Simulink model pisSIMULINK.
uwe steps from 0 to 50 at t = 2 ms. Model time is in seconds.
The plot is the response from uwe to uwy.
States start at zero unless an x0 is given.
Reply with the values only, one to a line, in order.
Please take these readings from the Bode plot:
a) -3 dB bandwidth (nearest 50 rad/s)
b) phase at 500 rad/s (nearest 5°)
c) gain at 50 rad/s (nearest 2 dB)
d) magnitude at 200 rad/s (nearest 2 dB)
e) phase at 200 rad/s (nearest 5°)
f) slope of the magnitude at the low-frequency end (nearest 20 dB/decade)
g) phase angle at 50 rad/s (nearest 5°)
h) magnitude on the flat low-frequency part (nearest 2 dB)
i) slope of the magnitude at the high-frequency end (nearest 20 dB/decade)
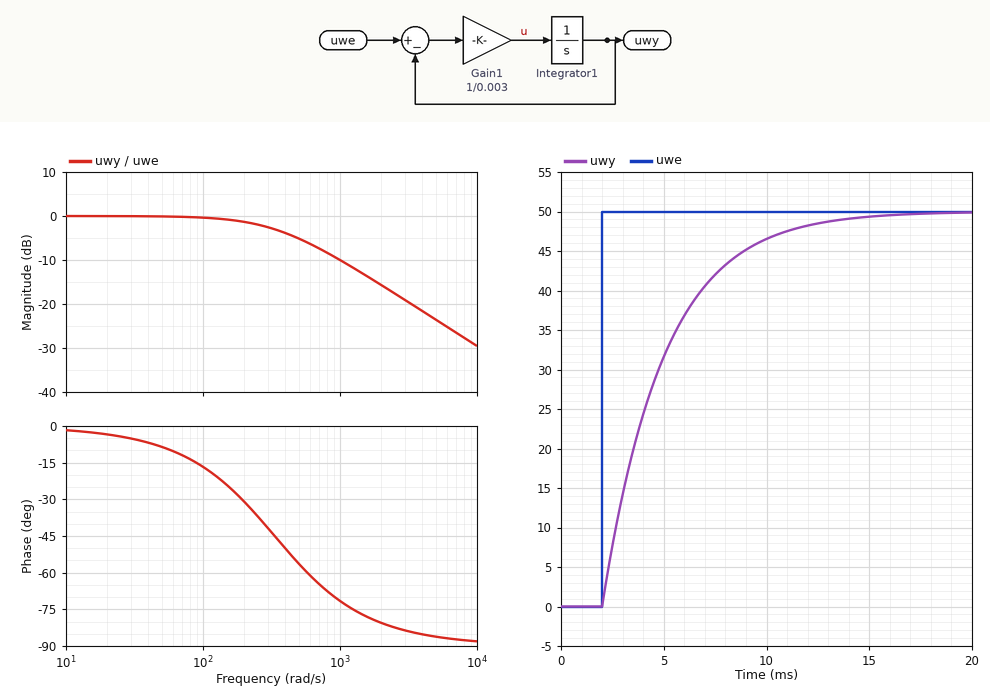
350 rad/s
-55°
0 dB
-2 dB
-30°
0 dB/decade
-10°
0 dB
-20 dB/decade
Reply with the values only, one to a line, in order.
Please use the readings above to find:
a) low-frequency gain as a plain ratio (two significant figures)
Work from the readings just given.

1.0
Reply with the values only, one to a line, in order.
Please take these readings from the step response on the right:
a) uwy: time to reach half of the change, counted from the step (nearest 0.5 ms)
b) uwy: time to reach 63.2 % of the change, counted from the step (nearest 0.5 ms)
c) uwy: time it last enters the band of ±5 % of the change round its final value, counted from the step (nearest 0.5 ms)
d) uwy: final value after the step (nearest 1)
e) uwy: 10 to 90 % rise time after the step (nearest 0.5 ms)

2.0 ms
3.0 ms
9.0 ms
50
6.5 ms
